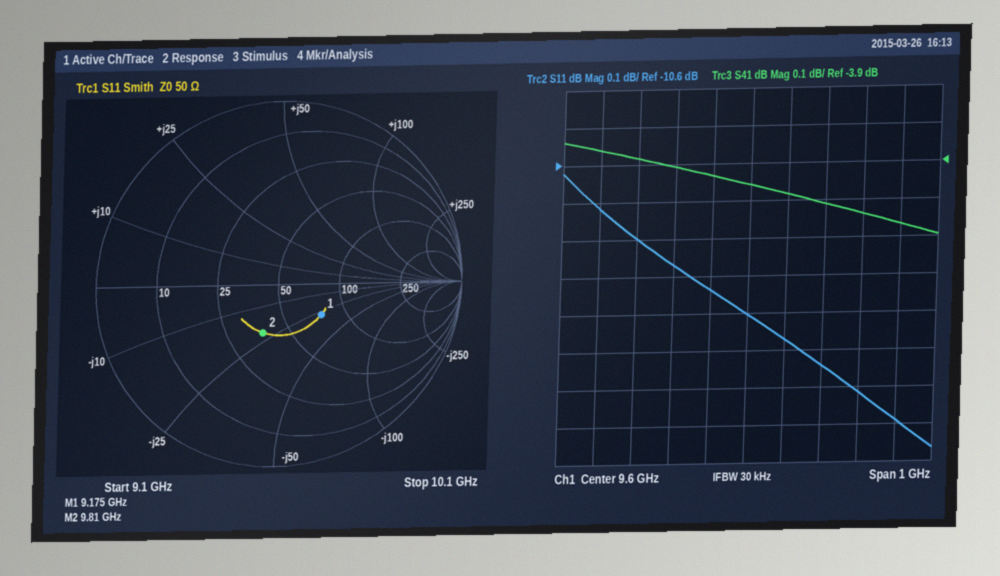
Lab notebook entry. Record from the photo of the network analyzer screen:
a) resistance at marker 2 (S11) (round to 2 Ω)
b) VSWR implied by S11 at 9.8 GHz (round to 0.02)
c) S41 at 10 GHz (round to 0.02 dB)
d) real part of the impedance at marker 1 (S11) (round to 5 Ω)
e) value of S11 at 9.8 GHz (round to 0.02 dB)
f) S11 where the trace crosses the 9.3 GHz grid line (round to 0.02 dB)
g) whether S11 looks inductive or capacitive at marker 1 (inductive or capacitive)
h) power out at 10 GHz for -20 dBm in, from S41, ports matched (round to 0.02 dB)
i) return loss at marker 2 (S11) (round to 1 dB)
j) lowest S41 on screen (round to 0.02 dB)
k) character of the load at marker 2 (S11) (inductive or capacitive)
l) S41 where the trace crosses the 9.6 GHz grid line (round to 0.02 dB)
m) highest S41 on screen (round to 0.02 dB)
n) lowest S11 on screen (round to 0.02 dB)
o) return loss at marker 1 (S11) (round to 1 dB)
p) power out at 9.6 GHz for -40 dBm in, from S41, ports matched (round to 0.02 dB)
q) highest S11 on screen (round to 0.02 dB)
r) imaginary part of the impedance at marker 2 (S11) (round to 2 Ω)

38 Ω
1.76
-4.06 dB
75 Ω
-11.14 dB
-10.80 dB
capacitive
-24.06 dBm
11 dB
-4.10 dB
capacitive
-3.96 dB
-3.84 dB
-11.36 dB
11 dB
-43.96 dBm
-10.62 dB
-22 Ω
